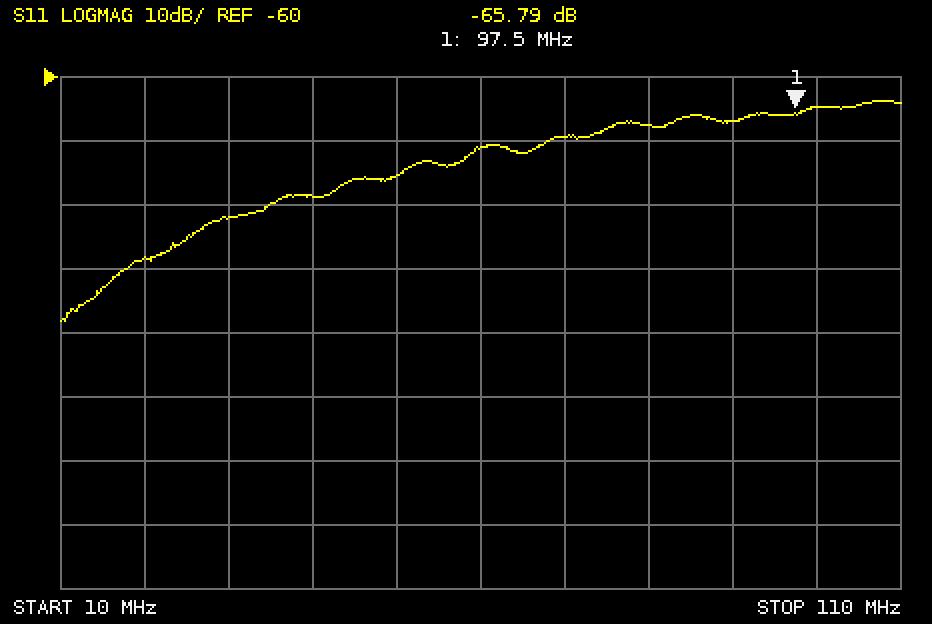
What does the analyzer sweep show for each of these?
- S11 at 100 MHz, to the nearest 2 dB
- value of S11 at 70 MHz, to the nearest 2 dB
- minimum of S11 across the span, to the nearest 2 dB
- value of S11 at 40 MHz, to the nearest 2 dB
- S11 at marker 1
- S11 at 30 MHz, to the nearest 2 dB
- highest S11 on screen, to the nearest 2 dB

-64 dB
-70 dB
-98 dB
-78 dB
-65.79 dB
-82 dB
-64 dB
